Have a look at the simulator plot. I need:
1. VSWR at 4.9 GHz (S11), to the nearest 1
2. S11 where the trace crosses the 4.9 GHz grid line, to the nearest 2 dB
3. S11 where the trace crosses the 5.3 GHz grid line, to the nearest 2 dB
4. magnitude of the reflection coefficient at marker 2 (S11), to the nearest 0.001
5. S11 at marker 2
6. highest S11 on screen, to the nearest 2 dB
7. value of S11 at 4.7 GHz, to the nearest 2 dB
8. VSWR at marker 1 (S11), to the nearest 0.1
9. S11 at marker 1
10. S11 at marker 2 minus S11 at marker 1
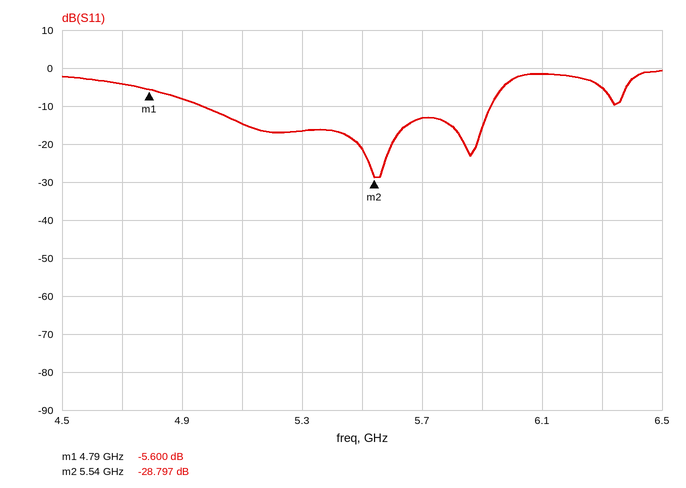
2
-8 dB
-16 dB
0.036
-28.797 dB
0 dB
-4 dB
3.2
-5.600 dB
-23.197 dB
